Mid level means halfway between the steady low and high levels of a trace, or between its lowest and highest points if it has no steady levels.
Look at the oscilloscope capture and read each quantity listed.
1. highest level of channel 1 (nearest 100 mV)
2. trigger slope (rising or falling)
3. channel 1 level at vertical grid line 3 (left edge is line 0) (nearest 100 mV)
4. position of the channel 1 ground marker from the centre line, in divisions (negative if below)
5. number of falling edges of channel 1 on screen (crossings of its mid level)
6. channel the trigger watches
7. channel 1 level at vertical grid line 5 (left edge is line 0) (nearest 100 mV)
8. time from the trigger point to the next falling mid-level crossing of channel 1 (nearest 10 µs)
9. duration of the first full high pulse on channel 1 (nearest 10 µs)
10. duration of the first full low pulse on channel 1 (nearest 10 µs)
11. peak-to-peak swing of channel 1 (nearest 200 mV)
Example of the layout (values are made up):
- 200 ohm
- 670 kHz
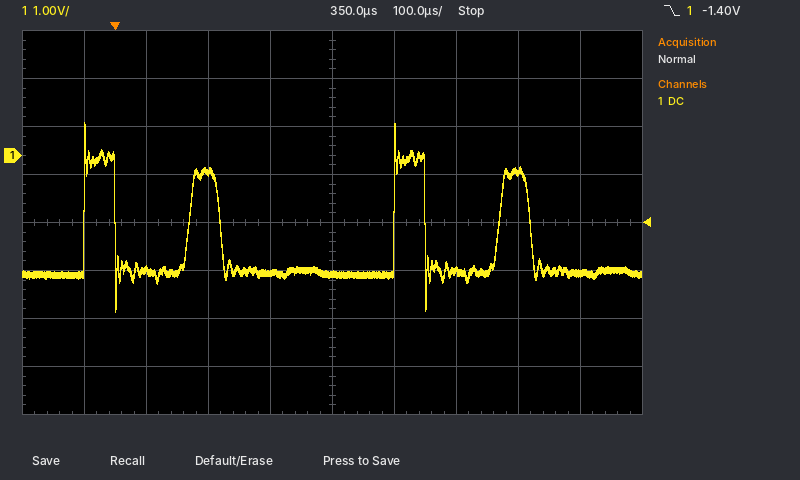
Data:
- 700 mV
- falling
- -300 mV
- +1.4 div
- 4
- channel 1
- -2.5 V
- 170 µs
- 50 µs
- 120 µs
- 4.0 V
